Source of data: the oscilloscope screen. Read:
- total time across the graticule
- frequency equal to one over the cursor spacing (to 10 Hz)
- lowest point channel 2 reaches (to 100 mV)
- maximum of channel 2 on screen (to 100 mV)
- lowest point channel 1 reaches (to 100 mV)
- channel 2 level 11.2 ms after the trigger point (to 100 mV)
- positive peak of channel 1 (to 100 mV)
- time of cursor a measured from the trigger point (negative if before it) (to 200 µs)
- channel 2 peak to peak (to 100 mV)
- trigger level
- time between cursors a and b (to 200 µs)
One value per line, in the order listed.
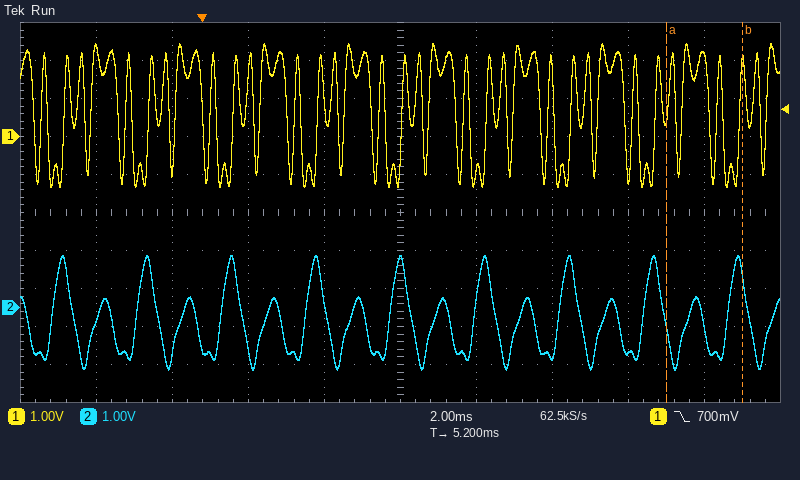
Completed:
20 ms
500 Hz
-1.6 V
1.4 V
-1.3 V
-1.2 V
2.4 V
+12.2 ms
3.0 V
700 mV
2.0 ms
